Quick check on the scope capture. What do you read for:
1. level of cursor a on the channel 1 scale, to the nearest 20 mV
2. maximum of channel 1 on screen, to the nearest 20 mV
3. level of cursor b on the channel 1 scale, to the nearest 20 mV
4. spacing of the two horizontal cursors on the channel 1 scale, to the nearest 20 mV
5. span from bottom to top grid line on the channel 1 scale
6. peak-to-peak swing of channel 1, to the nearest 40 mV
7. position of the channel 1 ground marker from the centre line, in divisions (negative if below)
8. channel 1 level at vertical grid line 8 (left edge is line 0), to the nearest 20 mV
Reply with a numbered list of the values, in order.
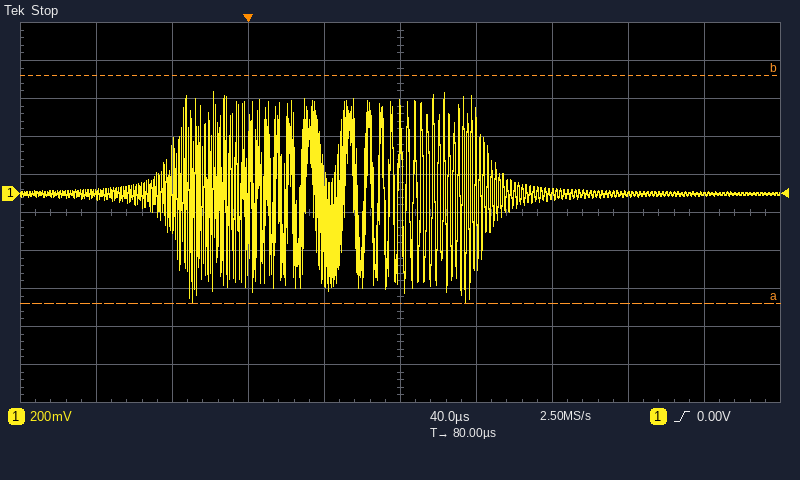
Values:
1. -580 mV
2. 540 mV
3. 620 mV
4. 1.20 V
5. 2 V
6. 1.12 V
7. +0.5 div
8. 0 mV
